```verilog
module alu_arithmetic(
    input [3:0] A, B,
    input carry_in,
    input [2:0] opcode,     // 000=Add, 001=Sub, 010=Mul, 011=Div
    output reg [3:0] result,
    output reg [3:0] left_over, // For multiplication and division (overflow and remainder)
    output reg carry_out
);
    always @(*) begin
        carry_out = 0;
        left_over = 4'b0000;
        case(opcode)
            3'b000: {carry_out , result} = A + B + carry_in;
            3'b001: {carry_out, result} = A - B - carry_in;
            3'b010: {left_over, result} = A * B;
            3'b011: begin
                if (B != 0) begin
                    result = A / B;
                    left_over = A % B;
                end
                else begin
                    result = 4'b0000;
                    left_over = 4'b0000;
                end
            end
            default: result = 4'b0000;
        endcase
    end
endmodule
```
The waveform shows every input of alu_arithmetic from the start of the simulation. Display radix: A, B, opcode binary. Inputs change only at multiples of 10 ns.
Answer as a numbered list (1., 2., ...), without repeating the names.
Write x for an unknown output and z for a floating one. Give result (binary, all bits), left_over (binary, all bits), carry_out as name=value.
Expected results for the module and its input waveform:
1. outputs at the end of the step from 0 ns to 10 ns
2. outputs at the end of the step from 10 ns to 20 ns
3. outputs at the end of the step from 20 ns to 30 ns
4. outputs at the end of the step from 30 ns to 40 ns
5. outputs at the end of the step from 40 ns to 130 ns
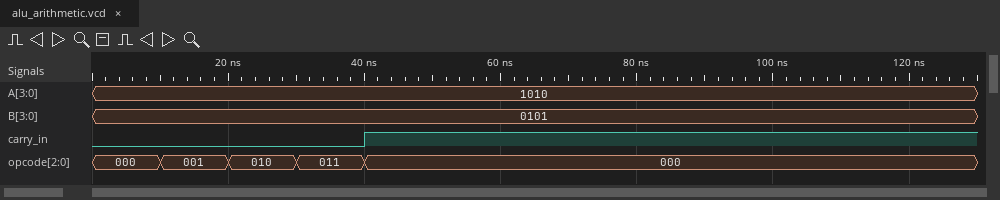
1. result=1111, left_over=0000, carry_out=0
2. result=0101, left_over=0000, carry_out=0
3. result=0010, left_over=0011, carry_out=0
4. result=0010, left_over=0000, carry_out=0
5. result=0000, left_over=0000, carry_out=1
